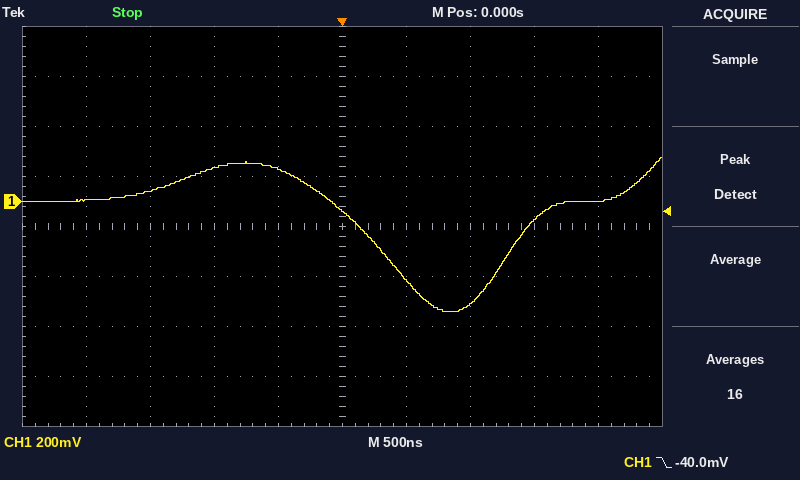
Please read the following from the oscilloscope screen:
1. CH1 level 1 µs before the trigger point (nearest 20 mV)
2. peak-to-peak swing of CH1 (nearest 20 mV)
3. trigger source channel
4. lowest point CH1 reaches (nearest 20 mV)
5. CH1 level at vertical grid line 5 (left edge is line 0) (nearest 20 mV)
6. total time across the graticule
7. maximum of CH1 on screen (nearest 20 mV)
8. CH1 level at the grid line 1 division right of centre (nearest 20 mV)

140 mV
620 mV
CH1
-440 mV
-40 mV
5 µs
180 mV
-320 mV
